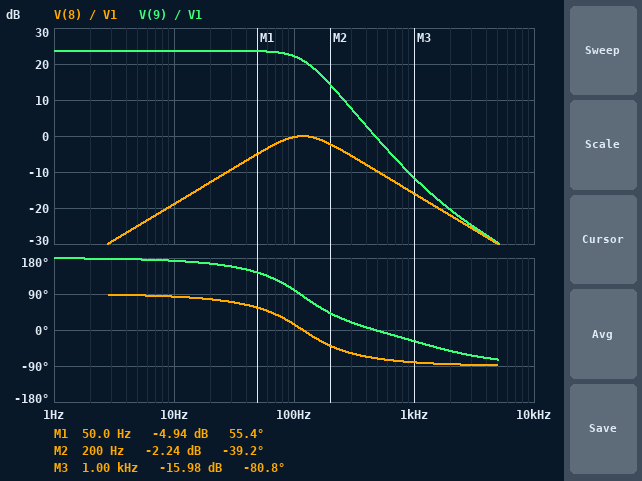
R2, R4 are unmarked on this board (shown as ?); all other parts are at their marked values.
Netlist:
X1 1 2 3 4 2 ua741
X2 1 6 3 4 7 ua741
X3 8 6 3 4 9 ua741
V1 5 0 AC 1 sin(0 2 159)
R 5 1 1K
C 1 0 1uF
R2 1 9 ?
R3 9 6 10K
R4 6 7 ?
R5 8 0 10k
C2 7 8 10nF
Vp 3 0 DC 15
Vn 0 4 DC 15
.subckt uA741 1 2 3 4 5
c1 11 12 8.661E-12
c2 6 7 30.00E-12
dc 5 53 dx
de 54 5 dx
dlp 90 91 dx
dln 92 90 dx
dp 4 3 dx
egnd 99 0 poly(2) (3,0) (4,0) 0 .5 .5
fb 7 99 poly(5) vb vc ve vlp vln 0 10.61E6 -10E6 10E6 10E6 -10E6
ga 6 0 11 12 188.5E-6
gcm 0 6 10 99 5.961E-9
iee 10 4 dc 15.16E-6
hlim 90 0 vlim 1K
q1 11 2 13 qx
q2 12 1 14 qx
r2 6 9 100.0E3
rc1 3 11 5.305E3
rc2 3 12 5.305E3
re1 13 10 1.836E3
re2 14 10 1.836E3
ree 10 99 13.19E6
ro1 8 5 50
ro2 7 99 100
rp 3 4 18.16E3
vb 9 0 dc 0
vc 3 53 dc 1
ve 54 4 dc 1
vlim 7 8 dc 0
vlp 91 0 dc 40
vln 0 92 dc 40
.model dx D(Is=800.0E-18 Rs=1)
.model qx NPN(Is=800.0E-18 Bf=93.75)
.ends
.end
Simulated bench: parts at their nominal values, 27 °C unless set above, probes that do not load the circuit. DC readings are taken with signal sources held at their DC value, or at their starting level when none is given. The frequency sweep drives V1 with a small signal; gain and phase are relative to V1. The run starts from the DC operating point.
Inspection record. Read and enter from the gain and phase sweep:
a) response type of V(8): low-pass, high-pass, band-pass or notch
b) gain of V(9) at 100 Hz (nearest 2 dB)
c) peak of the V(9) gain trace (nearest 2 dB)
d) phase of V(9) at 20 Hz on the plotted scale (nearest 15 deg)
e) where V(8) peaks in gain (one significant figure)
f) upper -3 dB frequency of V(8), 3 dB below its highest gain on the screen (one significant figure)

band-pass
22 dB
24 dB
165 deg
100 Hz
200 Hz
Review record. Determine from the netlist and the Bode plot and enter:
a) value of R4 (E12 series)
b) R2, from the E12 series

12 kΩ
15 kΩ
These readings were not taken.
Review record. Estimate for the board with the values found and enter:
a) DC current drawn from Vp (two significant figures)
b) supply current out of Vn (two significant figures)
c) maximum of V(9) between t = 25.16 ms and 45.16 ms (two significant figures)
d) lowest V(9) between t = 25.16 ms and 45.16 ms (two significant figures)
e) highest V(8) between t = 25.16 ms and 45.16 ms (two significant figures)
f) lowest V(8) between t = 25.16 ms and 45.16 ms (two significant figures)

5.0 mA
5.0 mA
12 V
-12 V
1.7 V
-1.7 V
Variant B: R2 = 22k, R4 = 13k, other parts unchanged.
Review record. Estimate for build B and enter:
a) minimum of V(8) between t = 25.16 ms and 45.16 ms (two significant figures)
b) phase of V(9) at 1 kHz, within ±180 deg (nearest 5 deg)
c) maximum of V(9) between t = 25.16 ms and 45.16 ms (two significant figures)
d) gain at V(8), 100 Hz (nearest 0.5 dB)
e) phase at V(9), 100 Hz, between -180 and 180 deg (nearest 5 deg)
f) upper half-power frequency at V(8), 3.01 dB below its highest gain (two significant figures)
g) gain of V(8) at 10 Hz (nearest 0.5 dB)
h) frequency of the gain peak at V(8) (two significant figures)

-1.6 V
-30 deg
11 V
0 dB
80 deg
200 Hz
-15.0 dB
94 Hz
